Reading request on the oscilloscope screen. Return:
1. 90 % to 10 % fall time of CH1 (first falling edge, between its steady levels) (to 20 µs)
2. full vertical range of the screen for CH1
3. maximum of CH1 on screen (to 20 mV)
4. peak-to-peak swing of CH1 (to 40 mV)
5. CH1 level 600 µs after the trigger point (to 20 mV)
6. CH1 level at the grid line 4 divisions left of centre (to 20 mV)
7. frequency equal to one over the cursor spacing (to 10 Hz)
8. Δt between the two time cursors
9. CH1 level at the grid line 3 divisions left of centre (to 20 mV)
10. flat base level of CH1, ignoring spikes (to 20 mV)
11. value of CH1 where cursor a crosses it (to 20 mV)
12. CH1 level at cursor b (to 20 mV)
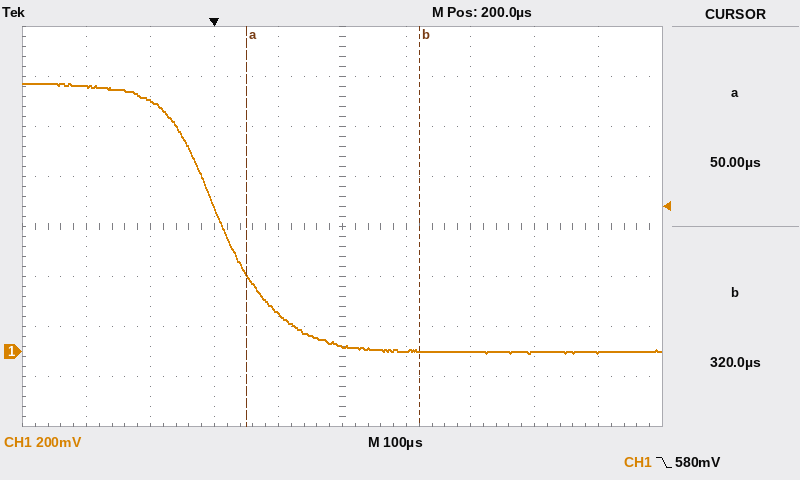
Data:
200 µs
1.6 V
1.08 V
1.08 V
0 mV
1.06 V
3.70 kHz
270 µs
1.00 V
0 mV
300 mV
0 mV
